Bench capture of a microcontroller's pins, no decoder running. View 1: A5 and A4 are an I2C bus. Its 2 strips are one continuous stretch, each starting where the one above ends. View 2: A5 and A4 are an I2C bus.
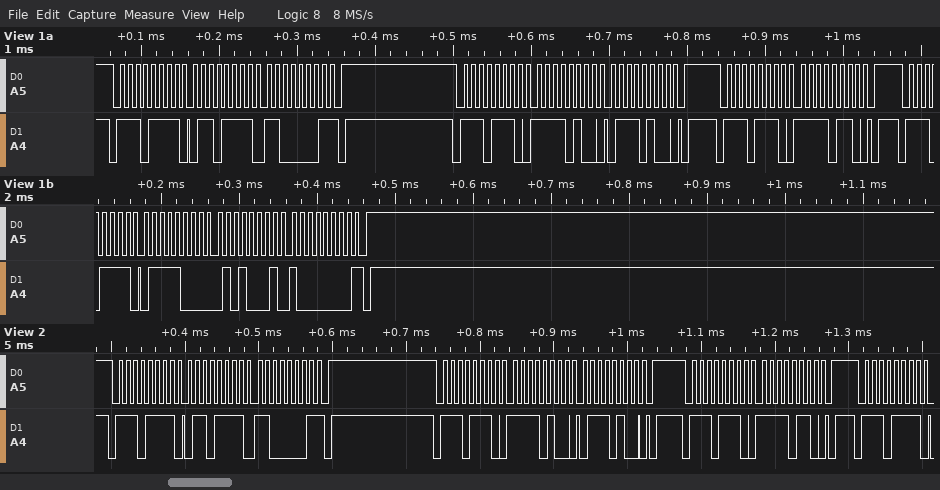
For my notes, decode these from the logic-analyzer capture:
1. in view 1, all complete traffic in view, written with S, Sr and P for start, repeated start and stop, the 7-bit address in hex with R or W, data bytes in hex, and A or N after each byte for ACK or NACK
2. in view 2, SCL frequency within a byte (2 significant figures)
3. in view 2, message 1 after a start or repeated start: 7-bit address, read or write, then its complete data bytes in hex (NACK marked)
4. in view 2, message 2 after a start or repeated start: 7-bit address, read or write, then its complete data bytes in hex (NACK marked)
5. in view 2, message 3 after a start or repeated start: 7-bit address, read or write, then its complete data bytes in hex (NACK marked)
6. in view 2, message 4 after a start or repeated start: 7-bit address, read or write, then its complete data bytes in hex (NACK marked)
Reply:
S 77R A 6F A C1 N P S 77W A F4 A 74 A P S 77W A F6 A P S 77R A 78 A 51 A 80 N P
100 kHz
0x77 read: 6F C1 NACK
0x77 write: F4 74
0x77 write: F6
0x77 read
